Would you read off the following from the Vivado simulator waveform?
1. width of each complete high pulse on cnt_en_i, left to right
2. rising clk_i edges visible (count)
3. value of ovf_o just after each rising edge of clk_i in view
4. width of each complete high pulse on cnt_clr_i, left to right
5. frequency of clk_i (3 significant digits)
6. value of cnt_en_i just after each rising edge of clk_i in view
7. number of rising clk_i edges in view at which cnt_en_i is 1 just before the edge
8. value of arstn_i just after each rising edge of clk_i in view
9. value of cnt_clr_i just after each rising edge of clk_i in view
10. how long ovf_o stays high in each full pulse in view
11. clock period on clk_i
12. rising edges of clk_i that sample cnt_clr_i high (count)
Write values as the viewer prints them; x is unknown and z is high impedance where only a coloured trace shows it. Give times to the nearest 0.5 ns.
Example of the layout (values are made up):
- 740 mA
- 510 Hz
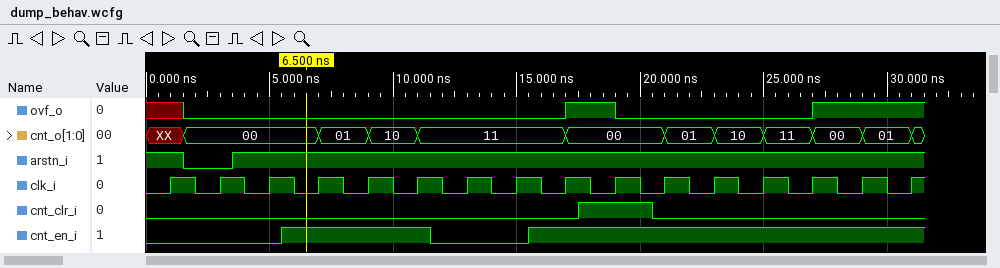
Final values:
- 6 ns
- 16
- x 0 0 0 0 0 0 0 1 0 0 0 0 1 1 1
- 3 ns
- 500 MHz
- 0 0 0 1 1 1 0 0 1 1 1 1 1 1 1 1
- 11
- 1 0 1 1 1 1 1 1 1 1 1 1 1 1 1 1
- 0 0 0 0 0 0 0 0 0 1 0 0 0 0 0 0
- 2 ns
- 2 ns
- 1
